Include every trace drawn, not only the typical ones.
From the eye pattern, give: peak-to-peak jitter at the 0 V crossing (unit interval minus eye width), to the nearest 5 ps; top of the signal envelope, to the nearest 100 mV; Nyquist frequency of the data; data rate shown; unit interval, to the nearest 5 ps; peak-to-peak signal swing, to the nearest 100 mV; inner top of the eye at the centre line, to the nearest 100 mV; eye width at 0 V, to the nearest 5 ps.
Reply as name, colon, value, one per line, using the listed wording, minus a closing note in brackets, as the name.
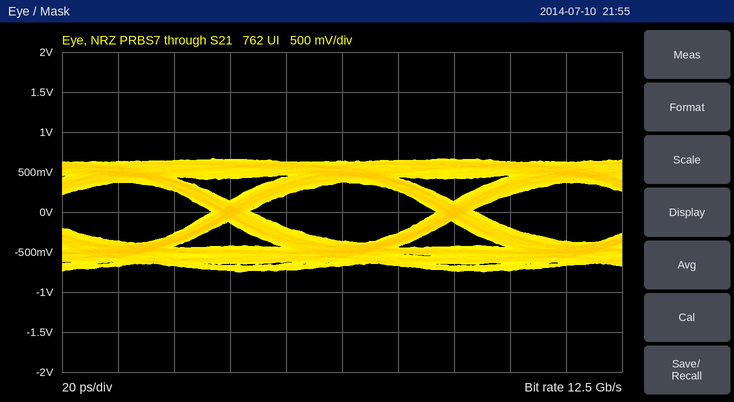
peak-to-peak jitter at the 0 V crossing (unit interval minus eye width), to the nearest 5 ps: 15 ps
top of the signal envelope, to the nearest 100 mV: 700 mV
Nyquist frequency of the data: 6.25 GHz
data rate shown: 12.5 Gb/s
unit interval, to the nearest 5 ps: 80 ps
peak-to-peak signal swing, to the nearest 100 mV: 1.4 V
inner top of the eye at the centre line, to the nearest 100 mV: 400 mV
eye width at 0 V, to the nearest 5 ps: 65 ps
